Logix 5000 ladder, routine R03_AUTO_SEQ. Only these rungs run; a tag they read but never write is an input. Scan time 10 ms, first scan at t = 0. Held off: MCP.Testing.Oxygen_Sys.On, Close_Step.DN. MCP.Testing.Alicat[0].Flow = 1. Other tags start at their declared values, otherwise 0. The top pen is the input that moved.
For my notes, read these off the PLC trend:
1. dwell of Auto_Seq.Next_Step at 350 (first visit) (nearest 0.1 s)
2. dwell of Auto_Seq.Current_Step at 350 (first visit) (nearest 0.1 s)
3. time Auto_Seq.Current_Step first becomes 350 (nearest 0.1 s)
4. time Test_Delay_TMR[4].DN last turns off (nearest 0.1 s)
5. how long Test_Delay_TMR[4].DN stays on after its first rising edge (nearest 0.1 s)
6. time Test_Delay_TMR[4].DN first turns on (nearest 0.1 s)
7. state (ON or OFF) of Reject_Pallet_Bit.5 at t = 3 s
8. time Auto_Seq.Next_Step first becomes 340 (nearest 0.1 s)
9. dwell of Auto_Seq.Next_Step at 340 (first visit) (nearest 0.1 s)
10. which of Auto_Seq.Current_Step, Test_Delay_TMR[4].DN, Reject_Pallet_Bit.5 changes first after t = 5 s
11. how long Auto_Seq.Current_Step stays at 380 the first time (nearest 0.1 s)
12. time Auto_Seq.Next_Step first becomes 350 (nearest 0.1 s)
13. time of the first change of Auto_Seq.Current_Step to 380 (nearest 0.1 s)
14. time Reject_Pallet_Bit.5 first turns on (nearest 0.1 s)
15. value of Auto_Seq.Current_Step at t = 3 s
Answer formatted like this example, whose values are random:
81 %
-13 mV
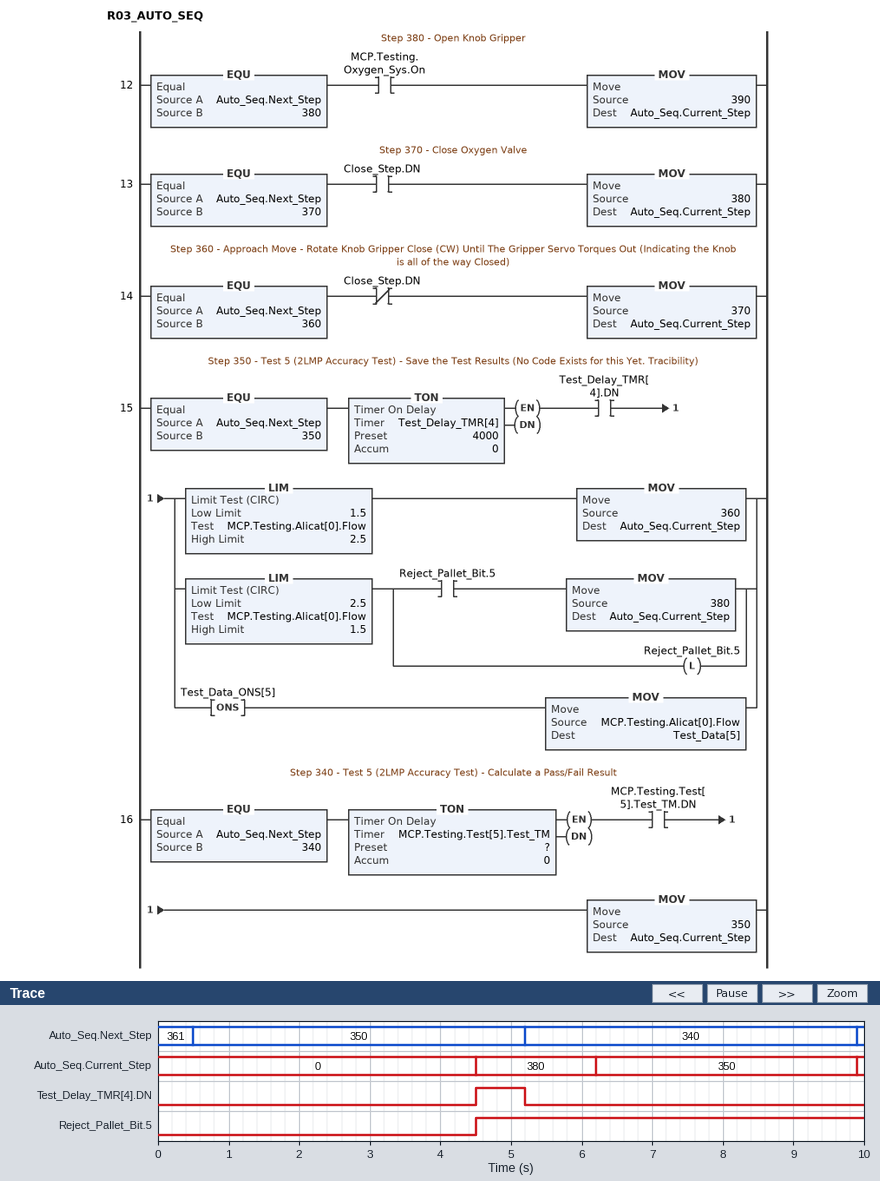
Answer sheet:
4.7 s
3.7 s
6.2 s
5.2 s
0.7 s
4.5 s
OFF
5.2 s
4.7 s
Test_Delay_TMR[4].DN
1.7 s
0.5 s
4.5 s
4.5 s
0
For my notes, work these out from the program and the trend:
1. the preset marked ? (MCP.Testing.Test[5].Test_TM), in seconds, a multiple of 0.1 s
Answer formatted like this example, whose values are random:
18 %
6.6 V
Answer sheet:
1.0 s
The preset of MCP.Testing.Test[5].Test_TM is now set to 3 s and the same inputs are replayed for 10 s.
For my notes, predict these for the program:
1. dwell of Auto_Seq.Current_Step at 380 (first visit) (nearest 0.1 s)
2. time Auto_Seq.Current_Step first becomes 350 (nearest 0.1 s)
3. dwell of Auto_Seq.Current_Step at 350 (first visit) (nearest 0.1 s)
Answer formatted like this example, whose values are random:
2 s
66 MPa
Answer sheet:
3.7 s
8.2 s
1.7 s
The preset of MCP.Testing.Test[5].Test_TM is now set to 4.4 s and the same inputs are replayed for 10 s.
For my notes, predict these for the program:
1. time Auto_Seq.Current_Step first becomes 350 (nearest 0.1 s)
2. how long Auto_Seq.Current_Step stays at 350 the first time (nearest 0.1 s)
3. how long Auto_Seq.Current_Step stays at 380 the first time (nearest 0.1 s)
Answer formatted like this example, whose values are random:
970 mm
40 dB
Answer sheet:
9.6 s
0.3 s
5.1 s
